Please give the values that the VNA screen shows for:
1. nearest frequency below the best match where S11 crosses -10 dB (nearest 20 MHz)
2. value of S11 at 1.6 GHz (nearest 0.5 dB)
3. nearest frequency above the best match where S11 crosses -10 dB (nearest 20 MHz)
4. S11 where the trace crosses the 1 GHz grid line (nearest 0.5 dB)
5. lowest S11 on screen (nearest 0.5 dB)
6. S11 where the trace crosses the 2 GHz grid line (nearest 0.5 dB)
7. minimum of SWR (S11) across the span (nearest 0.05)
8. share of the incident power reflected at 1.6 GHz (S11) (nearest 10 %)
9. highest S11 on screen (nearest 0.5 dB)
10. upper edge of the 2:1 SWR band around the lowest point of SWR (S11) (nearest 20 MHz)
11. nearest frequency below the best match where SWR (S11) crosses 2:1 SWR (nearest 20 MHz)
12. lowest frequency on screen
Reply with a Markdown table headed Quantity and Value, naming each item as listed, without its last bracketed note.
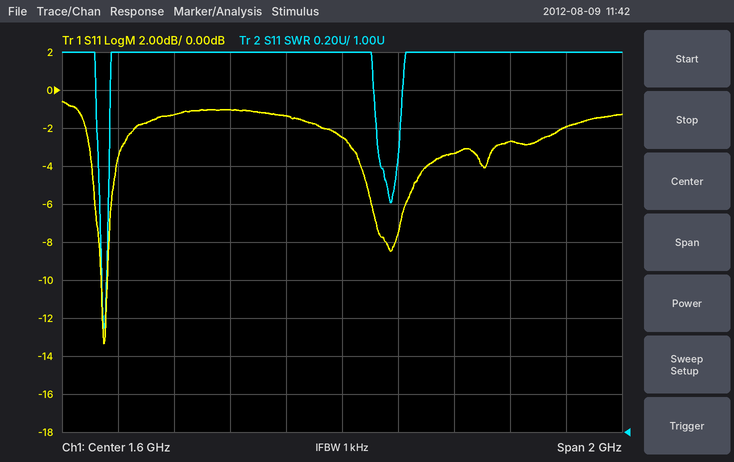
| Quantity | Value |
|---|---|
| nearest frequency below the best match where S11 crosses -10 dB | 740 MHz |
| value of S11 at 1.6 GHz | -2.5 dB |
| nearest frequency above the best match where S11 crosses -10 dB | 760 MHz |
| S11 where the trace crosses the 1 GHz grid line | -1.5 dB |
| lowest S11 on screen | -13.5 dB |
| S11 where the trace crosses the 2 GHz grid line | -3.5 dB |
| minimum of SWR (S11) across the span | 1.55 |
| share of the incident power reflected at 1.6 GHz (S11) | 60 % |
| highest S11 on screen | -0.5 dB |
| upper edge of the 2:1 SWR band around the lowest point of SWR (S11) | 760 MHz |
| nearest frequency below the best match where SWR (S11) crosses 2:1 SWR | 740 MHz |
| lowest frequency on screen | 600 MHz |
